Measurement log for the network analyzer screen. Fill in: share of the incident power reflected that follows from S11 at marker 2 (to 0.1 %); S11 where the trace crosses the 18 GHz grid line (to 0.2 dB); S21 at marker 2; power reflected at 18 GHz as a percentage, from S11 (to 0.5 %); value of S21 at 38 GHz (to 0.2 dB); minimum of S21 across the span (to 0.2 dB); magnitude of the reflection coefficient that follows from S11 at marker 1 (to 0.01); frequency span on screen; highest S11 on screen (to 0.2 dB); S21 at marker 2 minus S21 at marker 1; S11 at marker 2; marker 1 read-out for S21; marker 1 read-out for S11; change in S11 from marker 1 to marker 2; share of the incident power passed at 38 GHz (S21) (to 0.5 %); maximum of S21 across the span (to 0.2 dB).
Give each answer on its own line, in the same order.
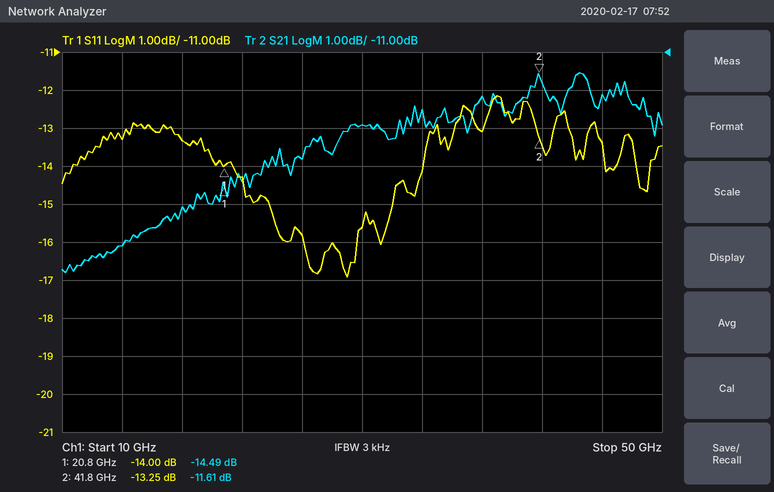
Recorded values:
4.7 %
-13.4 dB
-11.61 dB
4.5 %
-12.2 dB
-16.8 dB
0.20
40 GHz
-12.2 dB
2.88 dB
-13.25 dB
-14.49 dB
-14.00 dB
0.75 dB
6.0 %
-11.6 dB
